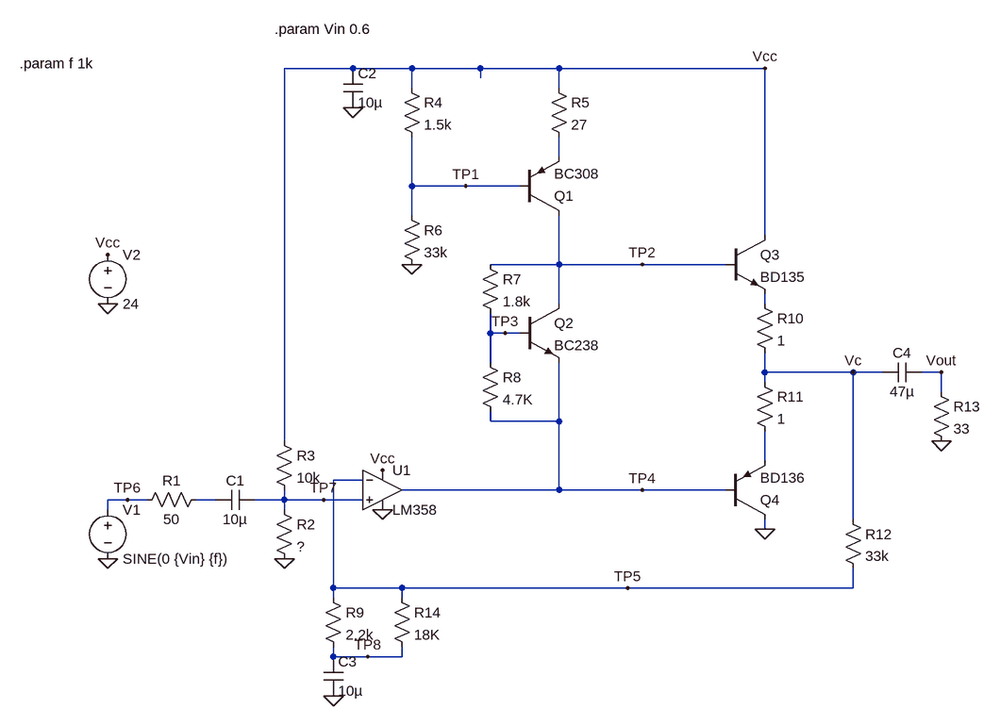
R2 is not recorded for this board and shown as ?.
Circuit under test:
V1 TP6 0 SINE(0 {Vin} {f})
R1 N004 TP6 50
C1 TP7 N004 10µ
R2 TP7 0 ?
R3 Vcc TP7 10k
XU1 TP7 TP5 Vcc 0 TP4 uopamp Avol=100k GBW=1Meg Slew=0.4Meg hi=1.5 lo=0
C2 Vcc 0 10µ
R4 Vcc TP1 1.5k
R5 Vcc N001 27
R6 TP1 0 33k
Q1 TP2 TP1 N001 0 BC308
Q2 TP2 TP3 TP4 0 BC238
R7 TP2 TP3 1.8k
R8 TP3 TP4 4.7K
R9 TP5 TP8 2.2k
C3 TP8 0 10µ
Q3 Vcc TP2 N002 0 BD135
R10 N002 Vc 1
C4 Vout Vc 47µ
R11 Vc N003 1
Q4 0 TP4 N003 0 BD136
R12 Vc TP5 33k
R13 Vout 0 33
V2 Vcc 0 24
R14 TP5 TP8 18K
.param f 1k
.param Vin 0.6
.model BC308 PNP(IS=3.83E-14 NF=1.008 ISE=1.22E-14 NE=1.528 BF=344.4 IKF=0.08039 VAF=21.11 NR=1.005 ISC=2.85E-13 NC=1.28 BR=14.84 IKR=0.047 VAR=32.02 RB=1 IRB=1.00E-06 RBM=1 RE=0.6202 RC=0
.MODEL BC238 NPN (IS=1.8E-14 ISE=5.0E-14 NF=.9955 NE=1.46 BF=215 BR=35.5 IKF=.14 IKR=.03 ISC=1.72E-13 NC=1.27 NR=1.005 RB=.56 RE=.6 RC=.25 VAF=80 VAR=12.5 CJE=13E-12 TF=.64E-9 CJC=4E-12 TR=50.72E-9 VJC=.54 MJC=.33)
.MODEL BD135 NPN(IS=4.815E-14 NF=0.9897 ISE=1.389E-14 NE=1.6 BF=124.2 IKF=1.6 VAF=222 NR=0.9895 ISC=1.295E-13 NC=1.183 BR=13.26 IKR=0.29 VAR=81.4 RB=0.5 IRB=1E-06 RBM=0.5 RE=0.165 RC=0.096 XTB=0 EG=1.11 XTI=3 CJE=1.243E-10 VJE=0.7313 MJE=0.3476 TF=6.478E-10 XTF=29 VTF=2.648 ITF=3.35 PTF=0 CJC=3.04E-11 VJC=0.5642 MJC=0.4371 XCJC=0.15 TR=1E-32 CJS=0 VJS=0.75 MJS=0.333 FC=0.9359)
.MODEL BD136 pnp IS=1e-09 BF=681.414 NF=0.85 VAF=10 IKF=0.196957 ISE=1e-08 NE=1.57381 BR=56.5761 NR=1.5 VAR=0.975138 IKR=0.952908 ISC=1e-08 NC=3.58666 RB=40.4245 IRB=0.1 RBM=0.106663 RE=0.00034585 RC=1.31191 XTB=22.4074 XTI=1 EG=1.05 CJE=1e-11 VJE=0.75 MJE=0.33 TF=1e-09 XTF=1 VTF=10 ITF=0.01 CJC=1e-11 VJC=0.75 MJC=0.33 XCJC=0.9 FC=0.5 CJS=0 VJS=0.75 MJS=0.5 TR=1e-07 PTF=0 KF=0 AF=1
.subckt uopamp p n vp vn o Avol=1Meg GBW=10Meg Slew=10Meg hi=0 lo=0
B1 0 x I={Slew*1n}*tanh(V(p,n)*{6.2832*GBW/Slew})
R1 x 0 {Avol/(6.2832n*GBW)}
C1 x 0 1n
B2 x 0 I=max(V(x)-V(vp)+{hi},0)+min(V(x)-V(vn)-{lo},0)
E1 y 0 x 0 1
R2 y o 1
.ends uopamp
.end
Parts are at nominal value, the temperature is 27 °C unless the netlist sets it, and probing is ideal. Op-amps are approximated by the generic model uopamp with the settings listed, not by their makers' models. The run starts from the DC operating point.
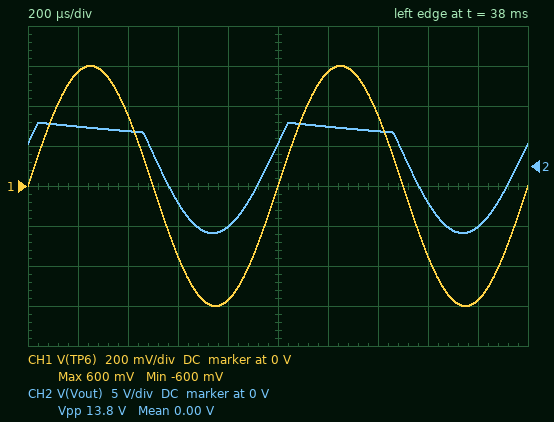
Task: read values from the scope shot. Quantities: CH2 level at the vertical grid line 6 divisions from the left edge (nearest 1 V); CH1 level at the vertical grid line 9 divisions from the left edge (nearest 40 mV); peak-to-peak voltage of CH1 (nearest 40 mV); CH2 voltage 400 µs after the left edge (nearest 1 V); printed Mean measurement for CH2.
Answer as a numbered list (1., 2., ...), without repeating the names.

1. 5 V
2. -560 mV
3. 1.20 V
4. 4 V
5. 0.00 V
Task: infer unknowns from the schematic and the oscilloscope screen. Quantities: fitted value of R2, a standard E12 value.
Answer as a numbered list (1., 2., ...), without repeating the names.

1. 33 kΩ
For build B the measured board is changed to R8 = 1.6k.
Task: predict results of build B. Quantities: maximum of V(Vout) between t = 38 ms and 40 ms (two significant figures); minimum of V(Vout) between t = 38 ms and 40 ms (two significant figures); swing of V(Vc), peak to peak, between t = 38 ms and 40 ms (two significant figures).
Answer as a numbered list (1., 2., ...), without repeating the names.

1. 5.6 V
2. -8.5 V
3. 14 V
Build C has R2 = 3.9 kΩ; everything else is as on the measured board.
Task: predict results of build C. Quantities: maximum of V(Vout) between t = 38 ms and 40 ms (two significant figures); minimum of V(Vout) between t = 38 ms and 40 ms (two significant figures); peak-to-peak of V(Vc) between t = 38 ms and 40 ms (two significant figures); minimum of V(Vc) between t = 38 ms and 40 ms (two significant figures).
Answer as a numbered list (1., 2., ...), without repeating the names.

1. 9.2 V
2. -6.9 V
3. 16 V
4. 710 mV
